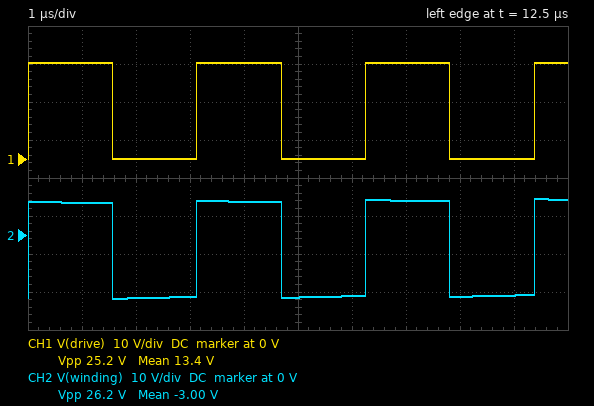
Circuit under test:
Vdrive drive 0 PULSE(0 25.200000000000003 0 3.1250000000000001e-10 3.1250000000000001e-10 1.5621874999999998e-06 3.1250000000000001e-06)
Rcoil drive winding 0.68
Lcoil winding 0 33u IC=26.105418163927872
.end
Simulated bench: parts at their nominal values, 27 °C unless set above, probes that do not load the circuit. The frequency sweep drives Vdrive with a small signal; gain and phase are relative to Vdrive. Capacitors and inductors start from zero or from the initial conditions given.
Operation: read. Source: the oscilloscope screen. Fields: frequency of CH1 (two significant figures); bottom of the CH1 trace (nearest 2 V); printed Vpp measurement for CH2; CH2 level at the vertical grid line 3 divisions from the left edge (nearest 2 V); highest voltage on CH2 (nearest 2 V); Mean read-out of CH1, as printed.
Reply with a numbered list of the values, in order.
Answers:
1. 320 kHz
2. 0 V
3. 26.2 V
4. -16 V
5. 10 V
6. 13.4 V
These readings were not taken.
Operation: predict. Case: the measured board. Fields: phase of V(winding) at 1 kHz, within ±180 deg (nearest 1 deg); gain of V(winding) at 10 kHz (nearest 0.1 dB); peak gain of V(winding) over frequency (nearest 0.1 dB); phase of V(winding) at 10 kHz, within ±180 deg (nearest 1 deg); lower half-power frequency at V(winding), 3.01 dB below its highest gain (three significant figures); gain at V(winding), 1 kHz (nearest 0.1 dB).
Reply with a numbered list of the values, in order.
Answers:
1. 73 deg
2. -0.4 dB
3. 0 dB
4. 18 deg
5. 3.28 kHz
6. -10.7 dB
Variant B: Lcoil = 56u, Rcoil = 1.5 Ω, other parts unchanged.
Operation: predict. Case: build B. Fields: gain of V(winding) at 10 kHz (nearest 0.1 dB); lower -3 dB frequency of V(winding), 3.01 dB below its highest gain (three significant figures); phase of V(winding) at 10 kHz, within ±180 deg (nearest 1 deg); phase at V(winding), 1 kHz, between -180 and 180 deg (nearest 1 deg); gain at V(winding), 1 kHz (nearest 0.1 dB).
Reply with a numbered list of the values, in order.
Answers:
1. -0.7 dB
2. 4.26 kHz
3. 23 deg
4. 77 deg
5. -12.8 dB
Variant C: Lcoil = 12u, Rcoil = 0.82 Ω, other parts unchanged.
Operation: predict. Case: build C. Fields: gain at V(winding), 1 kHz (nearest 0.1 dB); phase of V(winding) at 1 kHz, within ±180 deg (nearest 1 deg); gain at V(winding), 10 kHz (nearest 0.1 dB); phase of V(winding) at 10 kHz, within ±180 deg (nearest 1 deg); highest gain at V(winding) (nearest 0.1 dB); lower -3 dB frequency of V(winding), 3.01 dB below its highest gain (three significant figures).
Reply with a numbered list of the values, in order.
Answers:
1. -20.8 dB
2. 85 deg
3. -3.4 dB
4. 47 deg
5. 0 dB
6. 10.9 kHz
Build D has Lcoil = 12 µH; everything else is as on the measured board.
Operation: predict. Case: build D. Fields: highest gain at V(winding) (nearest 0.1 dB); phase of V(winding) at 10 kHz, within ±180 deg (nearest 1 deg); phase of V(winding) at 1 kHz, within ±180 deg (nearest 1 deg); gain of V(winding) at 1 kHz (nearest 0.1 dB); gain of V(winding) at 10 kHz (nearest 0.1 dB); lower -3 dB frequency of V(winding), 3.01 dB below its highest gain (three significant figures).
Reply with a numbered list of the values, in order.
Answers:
1. 0 dB
2. 42 deg
3. 84 deg
4. -19.2 dB
5. -2.6 dB
6. 9.02 kHz
